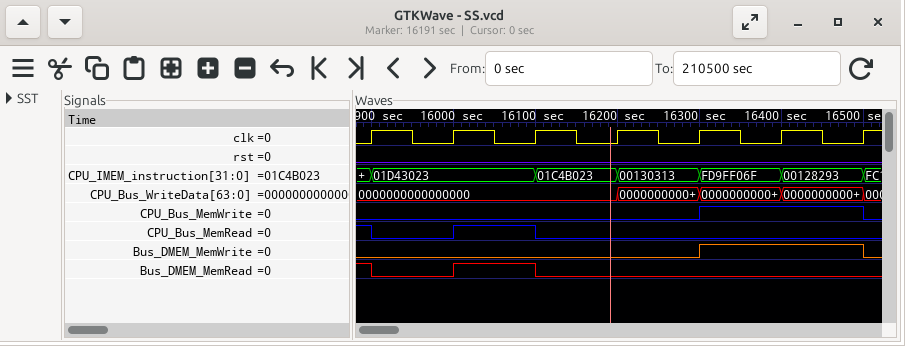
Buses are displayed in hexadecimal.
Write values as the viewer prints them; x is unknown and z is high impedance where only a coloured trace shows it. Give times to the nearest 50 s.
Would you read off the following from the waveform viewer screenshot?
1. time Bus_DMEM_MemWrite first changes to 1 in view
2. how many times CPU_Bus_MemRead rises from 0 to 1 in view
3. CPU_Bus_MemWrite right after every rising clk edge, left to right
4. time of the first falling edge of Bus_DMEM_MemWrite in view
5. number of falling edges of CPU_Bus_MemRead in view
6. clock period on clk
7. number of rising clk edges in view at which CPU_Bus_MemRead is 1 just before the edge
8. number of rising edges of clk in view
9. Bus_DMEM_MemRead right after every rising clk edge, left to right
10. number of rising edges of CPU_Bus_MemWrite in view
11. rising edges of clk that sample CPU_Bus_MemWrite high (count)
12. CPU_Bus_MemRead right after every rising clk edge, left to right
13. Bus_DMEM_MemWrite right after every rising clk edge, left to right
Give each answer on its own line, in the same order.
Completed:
16300 s
1
0 0 0 0 1 1 0
16500 s
2
100 s
2
7
0 1 0 0 0 0 0
1
2
0 1 0 0 0 0 0
0 0 0 0 1 1 0
